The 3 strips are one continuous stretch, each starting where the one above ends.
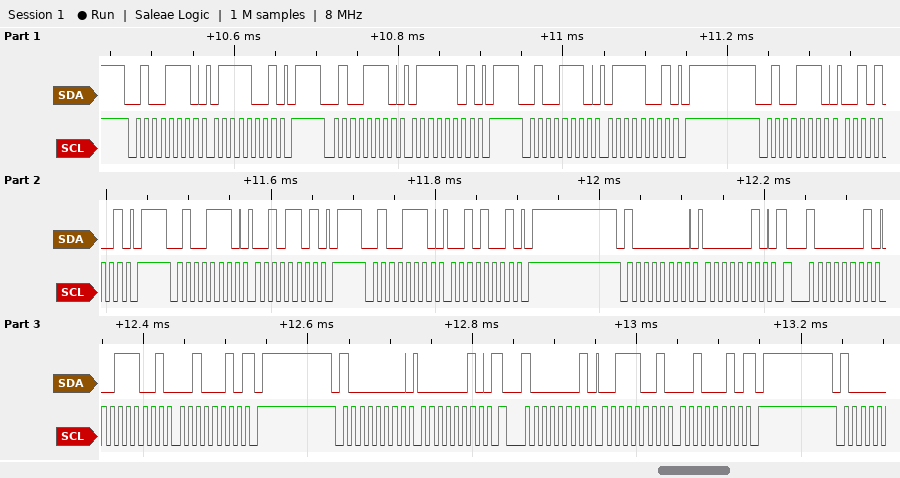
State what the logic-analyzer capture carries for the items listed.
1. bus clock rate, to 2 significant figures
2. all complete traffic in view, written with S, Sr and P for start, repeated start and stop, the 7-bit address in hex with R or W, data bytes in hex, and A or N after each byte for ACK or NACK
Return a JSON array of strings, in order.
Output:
["100 kHz", "S 27W A 79 A P S 27W A 7D A P S 27W A 79 A P S 27W A 29 A P S 27W A 2D A P S 27W A 29 A P S 40W A 02 A Sr 40R A 39 A 22 N P S 40W A 02 A Sr 40R A 39 A 22 N P"]
